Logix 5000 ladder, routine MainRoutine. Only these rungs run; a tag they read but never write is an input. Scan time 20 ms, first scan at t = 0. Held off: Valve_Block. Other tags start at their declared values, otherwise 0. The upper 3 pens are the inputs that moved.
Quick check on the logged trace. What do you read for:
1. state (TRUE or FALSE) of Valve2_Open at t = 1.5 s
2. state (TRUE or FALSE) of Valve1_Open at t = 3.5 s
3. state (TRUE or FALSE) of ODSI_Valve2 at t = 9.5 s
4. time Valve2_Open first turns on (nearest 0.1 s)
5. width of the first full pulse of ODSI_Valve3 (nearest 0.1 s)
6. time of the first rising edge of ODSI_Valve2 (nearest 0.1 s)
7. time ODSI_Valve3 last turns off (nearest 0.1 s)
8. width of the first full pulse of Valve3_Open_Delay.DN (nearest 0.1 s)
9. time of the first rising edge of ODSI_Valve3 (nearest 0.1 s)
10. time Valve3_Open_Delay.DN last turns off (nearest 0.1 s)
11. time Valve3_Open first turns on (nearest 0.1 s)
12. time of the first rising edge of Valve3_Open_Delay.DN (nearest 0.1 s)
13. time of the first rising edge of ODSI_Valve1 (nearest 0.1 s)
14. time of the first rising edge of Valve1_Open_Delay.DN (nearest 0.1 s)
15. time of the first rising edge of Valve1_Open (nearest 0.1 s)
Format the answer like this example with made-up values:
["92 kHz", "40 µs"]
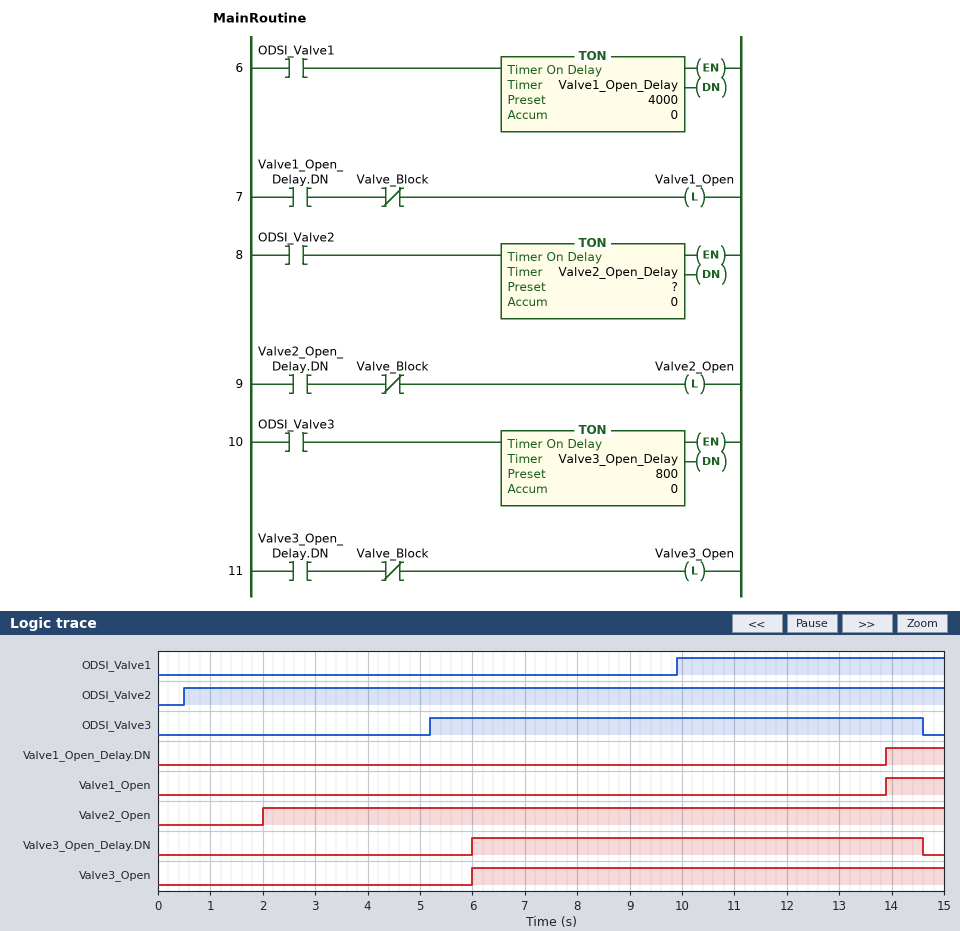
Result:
["FALSE", "FALSE", "TRUE", "2.0 s", "9.4 s", "0.5 s", "14.6 s", "8.6 s", "5.2 s", "14.6 s", "6.0 s", "6.0 s", "9.9 s", "13.9 s", "13.9 s"]
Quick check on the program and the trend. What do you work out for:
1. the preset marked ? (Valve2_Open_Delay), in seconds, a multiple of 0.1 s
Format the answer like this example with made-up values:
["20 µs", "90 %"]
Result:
["1.5 s"]
